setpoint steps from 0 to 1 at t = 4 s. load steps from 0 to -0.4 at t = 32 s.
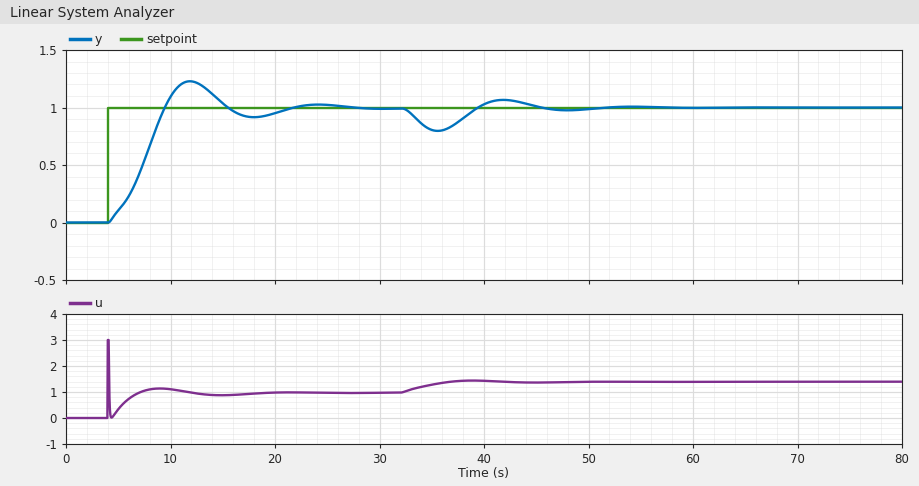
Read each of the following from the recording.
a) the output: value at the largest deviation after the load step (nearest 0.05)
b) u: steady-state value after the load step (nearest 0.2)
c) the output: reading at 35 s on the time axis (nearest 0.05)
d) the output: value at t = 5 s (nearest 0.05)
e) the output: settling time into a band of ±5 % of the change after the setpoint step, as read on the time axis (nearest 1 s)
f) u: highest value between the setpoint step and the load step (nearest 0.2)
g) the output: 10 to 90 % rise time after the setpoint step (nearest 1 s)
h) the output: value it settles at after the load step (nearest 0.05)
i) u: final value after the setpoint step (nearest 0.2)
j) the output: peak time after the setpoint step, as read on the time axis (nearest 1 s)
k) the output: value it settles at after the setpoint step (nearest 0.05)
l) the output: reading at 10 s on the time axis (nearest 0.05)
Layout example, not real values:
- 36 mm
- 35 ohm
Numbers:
- 0.80
- 1.4
- 0.80
- 0.10
- 20 s
- 3.0
- 4 s
- 1.00
- 1.0
- 12 s
- 1.00
- 1.10
